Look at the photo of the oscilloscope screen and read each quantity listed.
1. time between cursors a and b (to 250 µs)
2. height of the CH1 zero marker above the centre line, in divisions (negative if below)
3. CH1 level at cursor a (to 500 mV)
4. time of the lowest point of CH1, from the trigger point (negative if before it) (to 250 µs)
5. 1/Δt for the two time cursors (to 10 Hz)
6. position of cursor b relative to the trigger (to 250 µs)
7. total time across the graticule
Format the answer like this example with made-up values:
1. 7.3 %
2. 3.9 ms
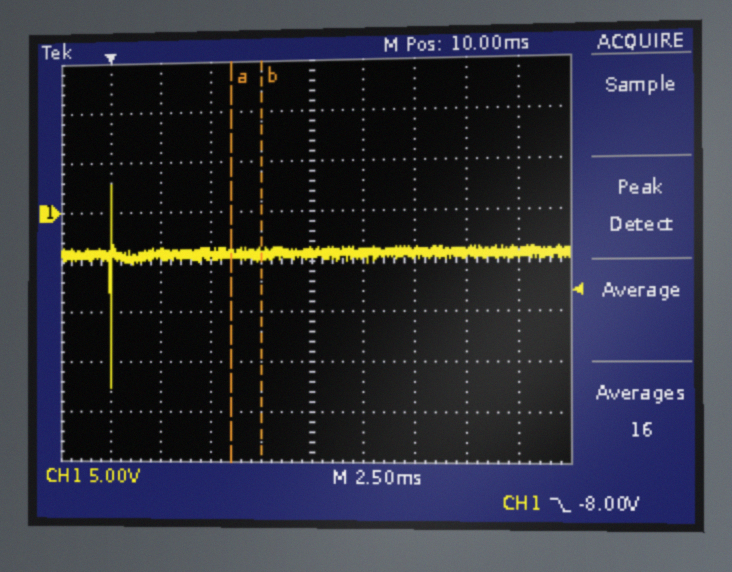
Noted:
1. 1.50 ms
2. +1.0 div
3. -4.0 V
4. 0.00 ms
5. 670 Hz
6. +7.50 ms
7. 25 ms
